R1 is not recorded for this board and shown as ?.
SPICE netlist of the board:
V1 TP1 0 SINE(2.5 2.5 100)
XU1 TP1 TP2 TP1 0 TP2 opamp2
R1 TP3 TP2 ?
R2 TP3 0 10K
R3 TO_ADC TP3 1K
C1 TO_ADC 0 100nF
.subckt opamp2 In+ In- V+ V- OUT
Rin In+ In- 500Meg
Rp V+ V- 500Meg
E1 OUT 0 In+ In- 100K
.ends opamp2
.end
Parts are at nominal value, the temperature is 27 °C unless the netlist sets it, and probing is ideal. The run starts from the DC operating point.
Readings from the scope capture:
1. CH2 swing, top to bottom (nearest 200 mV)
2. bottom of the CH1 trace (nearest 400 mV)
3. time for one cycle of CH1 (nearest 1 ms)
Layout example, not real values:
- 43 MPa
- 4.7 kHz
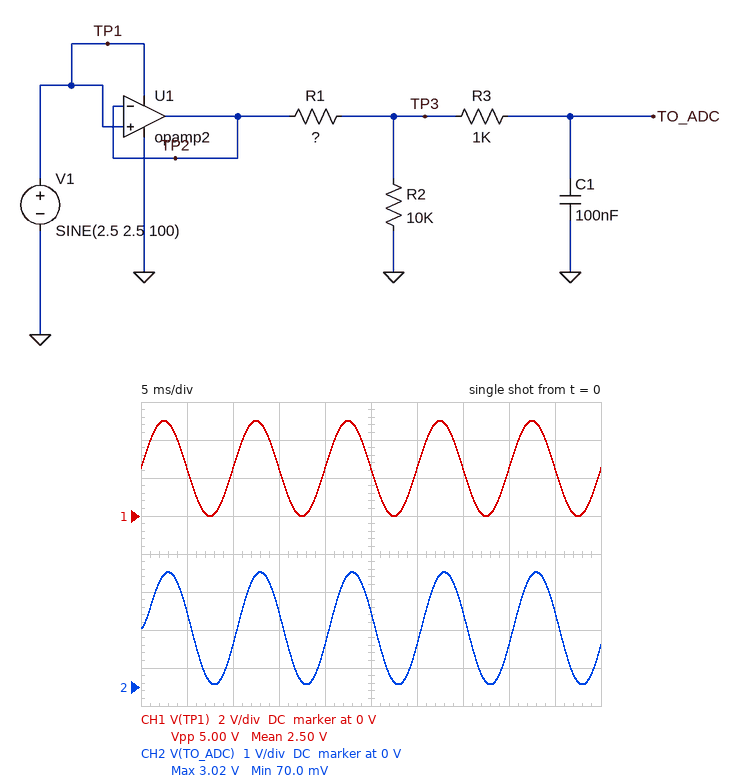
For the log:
- 3.0 V
- 0 V
- 10 ms
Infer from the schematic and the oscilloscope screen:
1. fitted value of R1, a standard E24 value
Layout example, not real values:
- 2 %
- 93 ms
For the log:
- 6.2 kΩ
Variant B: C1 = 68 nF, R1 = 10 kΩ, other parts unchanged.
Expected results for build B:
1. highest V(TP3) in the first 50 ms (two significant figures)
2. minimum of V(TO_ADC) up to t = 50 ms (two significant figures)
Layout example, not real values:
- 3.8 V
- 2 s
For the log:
- 2.5 V
- 39 mV
